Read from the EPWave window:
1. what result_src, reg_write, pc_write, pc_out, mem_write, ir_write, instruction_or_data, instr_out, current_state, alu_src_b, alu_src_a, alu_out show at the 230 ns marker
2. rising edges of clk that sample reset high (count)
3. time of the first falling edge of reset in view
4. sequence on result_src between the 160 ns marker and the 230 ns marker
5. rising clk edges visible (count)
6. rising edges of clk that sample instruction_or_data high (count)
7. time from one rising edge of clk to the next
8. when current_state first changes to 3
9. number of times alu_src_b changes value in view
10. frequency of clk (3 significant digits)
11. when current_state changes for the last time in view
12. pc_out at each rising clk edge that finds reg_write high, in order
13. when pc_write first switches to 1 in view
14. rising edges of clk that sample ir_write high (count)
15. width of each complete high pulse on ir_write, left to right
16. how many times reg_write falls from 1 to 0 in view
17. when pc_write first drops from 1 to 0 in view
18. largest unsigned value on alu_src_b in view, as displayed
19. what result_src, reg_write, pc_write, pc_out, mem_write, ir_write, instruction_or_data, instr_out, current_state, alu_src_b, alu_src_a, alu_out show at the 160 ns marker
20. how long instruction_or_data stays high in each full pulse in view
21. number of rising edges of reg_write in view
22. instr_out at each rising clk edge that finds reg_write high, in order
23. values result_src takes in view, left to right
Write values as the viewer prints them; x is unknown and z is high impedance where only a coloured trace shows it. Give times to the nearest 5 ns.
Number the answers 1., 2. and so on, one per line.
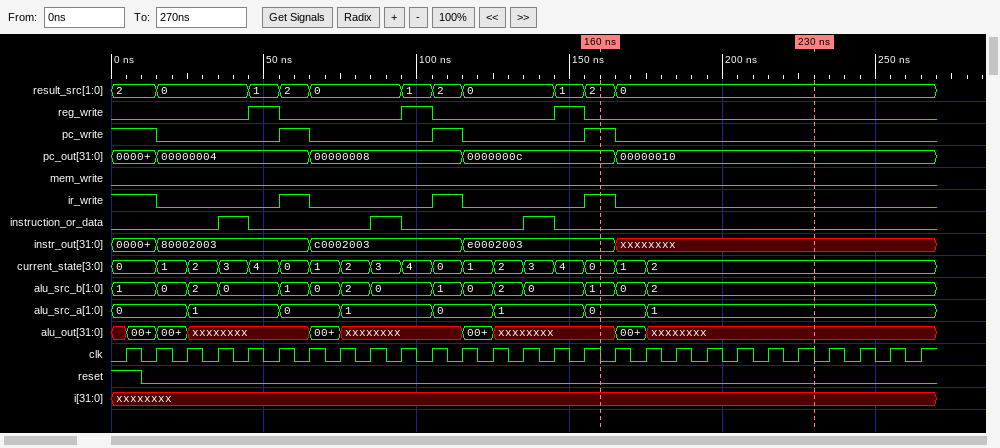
1. result_src=0, reg_write=0, pc_write=0, pc_out=00000010, mem_write=0, ir_write=0, instruction_or_data=0, instr_out=xxxxxxxx, current_state=2, alu_src_b=2, alu_src_a=1, alu_out=xxxxxxxx
2. 1
3. 10 ns
4. 2, 0
5. 27
6. 3
7. 10 ns
8. 35 ns
9. 14
10. 100 MHz
11. 175 ns
12. 00000004, 00000008, 0000000c
13. 55 ns
14. 5
15. 10 ns, 10 ns, 10 ns
16. 3
17. 15 ns
18. 2
19. result_src=2, reg_write=0, pc_write=1, pc_out=0000000c, mem_write=0, ir_write=1, instruction_or_data=0, instr_out=e0002003, current_state=0, alu_src_b=1, alu_src_a=0, alu_out=xxxxxxxx
20. 10 ns, 10 ns, 10 ns
21. 3
22. 80002003, c0002003, e0002003
23. 2, 0, 1, 2, 0, 1, 2, 0, 1, 2, 0
